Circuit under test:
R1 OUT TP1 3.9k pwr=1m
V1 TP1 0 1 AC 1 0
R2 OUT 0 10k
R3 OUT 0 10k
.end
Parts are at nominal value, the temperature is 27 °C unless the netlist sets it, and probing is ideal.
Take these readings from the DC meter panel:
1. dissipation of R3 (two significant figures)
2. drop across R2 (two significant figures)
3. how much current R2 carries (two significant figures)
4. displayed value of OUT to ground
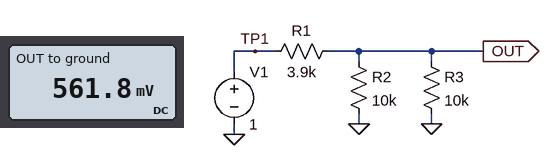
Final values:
32 µW
560 mV
56 µA
561.8 mV
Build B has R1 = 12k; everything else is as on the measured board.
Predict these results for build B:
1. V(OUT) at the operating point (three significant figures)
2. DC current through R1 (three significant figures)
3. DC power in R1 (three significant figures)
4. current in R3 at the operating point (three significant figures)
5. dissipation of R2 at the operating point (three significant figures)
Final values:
294 mV
58.8 µA
41.5 µW
29.4 µA
8.65 µW
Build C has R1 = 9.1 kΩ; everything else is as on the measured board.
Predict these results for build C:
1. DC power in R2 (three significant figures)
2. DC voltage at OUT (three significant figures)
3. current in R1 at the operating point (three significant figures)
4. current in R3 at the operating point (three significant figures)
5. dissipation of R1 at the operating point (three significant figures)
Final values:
12.6 µW
355 mV
70.9 µA
35.5 µA
45.8 µW
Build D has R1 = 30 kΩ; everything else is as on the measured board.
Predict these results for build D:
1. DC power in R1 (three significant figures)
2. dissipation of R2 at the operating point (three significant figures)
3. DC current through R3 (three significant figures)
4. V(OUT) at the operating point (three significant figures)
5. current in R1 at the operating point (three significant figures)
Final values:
24.5 µW
2.04 µW
14.3 µA
143 mV
28.6 µA
